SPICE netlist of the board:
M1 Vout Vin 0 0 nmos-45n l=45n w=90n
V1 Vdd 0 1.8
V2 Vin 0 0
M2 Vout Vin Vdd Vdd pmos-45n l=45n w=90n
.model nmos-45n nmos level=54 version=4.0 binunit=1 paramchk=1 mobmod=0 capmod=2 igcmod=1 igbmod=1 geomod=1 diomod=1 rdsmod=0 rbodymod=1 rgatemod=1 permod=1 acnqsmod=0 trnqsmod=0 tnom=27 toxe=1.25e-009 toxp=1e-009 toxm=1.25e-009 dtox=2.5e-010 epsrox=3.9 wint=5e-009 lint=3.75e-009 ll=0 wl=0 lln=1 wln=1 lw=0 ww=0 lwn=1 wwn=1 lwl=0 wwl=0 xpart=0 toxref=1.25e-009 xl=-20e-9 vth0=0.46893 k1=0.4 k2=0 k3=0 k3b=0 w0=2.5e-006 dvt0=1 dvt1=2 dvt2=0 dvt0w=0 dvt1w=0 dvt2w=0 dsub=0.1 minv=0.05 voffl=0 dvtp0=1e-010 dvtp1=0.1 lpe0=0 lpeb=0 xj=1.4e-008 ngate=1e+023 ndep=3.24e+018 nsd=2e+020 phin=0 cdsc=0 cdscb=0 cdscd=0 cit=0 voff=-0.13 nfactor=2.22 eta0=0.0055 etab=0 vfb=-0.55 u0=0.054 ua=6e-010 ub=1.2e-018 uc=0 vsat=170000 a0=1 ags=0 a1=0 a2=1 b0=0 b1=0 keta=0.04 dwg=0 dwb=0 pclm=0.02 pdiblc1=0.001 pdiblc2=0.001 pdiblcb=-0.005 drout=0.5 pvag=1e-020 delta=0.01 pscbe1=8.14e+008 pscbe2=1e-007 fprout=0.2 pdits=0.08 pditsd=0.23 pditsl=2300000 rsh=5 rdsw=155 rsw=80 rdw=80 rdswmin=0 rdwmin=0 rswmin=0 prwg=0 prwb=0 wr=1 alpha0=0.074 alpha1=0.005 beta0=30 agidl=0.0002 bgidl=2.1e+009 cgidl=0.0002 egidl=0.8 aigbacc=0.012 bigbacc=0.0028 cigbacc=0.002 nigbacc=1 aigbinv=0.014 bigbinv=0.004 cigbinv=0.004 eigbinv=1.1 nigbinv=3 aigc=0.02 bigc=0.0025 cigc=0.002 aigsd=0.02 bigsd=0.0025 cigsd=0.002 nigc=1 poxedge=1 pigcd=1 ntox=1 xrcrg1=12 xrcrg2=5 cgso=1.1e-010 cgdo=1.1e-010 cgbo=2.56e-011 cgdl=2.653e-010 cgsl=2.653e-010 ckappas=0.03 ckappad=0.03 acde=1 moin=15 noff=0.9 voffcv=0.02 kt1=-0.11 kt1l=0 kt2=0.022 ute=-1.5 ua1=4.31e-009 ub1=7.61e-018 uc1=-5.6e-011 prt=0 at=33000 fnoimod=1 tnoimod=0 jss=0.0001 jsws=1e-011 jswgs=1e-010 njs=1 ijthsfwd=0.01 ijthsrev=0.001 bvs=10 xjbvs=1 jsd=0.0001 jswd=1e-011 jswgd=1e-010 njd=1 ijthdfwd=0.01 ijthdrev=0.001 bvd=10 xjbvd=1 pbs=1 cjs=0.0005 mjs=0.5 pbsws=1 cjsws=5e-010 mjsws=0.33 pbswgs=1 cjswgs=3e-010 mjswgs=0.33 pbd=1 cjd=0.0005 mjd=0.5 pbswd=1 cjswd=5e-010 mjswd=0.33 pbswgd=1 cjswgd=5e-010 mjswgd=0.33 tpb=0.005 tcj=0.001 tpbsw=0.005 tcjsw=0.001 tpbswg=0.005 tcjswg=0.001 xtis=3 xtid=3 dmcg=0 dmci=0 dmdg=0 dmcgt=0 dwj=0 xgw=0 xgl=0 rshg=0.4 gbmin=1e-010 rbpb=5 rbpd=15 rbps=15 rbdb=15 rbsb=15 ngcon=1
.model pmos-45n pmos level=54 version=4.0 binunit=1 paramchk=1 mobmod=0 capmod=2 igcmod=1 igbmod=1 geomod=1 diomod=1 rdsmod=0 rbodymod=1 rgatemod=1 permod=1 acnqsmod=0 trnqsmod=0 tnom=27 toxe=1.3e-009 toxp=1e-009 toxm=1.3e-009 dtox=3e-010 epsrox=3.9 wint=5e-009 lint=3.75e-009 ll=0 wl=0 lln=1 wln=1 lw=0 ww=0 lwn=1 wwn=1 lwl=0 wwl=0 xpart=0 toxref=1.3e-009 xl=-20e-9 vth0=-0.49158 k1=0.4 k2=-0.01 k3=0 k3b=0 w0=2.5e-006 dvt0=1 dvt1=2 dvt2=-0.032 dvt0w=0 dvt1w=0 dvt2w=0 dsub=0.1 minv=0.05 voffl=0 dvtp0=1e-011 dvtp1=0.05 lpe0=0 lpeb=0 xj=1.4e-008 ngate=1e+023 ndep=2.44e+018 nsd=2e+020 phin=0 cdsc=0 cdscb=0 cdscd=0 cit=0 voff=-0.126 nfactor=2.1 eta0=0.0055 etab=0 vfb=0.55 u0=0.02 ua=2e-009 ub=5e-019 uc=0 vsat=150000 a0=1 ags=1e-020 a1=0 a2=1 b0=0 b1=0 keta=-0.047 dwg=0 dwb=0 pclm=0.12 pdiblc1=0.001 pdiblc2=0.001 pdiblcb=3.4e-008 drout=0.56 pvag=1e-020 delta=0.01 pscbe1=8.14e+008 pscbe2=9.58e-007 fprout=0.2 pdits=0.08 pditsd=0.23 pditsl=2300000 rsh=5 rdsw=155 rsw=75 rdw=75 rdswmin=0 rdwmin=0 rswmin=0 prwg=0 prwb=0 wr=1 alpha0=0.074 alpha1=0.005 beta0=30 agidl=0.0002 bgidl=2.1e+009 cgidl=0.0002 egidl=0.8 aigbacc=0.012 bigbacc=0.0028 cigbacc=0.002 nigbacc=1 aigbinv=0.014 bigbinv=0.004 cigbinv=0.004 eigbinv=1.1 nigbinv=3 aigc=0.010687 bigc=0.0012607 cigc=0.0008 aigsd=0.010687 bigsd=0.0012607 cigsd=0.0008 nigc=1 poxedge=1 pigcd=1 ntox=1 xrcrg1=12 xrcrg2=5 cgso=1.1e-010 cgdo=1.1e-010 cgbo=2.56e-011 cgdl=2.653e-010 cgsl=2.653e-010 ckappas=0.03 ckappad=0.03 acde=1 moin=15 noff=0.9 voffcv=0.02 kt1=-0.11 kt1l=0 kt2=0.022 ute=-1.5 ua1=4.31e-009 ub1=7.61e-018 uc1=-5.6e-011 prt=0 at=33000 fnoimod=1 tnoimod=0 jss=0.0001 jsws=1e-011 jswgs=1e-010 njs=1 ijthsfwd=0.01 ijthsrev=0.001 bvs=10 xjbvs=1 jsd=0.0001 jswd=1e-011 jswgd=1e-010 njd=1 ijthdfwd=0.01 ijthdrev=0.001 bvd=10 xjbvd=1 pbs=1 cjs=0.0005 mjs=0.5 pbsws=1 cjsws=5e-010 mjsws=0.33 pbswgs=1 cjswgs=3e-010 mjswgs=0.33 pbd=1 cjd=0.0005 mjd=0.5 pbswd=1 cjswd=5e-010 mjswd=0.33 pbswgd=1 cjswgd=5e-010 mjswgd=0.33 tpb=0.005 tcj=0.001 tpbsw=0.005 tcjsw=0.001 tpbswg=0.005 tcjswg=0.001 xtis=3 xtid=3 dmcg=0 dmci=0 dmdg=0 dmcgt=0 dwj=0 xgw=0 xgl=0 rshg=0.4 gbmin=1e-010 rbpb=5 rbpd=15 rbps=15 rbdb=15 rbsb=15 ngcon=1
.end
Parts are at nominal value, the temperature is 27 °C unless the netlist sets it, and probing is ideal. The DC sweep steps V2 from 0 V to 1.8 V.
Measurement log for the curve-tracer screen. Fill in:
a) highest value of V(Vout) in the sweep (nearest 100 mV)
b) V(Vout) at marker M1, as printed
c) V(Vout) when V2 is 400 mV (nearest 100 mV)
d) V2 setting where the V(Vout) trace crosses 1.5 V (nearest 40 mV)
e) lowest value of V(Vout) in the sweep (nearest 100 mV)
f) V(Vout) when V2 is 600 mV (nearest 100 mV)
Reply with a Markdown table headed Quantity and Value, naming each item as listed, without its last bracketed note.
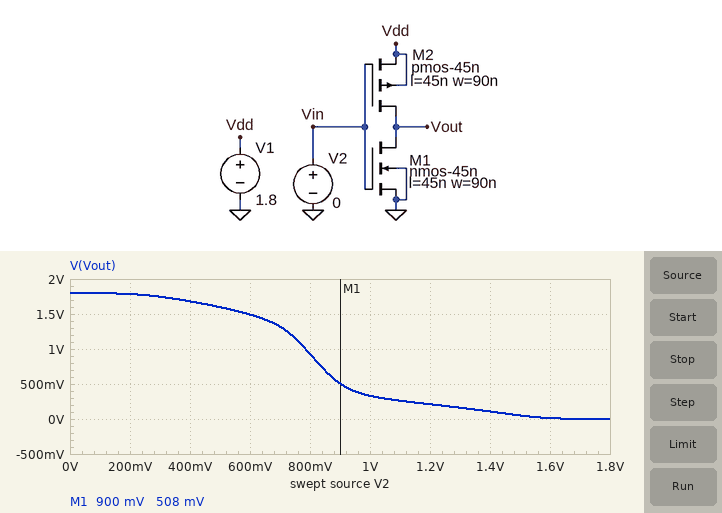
| Quantity | Value |
|---|---|
| highest value of V(Vout) in the sweep | 1.8 V |
| V(Vout) at marker M1, as printed | 508 mV |
| V(Vout) when V2 is 400 mV | 1.7 V |
| V2 setting where the V(Vout) trace crosses 1.5 V | 600 mV |
| lowest value of V(Vout) in the sweep | 0 V |
| V(Vout) when V2 is 600 mV | 1.5 V |
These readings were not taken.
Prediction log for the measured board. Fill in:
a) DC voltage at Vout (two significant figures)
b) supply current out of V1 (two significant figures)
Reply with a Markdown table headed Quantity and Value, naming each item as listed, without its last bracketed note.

| Quantity | Value |
|---|---|
| DC voltage at Vout | 1.8 V |
| supply current out of V1 | 1.8 µA |
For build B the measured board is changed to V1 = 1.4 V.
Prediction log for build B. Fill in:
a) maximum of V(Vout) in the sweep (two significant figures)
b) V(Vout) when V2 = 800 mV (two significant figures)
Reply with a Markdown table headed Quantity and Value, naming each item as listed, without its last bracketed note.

| Quantity | Value |
|---|---|
| maximum of V(Vout) in the sweep | 1.4 V |
| V(Vout) when V2 = 800 mV | 140 mV |
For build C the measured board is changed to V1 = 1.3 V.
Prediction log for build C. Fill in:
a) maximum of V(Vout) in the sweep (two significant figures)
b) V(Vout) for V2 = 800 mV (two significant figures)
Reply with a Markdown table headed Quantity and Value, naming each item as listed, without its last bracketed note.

| Quantity | Value |
|---|---|
| maximum of V(Vout) in the sweep | 1.3 V |
| V(Vout) for V2 = 800 mV | 70 mV |
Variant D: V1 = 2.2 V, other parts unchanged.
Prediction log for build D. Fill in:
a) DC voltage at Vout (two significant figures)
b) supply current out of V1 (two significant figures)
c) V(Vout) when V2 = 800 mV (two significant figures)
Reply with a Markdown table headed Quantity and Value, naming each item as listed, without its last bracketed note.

| Quantity | Value |
|---|---|
| DC voltage at Vout | 2.1 V |
| supply current out of V1 | 19 µA |
| V(Vout) when V2 = 800 mV | 1.6 V |
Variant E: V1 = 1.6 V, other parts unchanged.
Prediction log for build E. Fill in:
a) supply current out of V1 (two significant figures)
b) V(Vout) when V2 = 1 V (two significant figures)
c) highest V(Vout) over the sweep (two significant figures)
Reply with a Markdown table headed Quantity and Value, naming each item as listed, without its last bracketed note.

| Quantity | Value |
|---|---|
| supply current out of V1 | 230 nA |
| V(Vout) when V2 = 1 V | 160 mV |
| highest V(Vout) over the sweep | 1.6 V |
